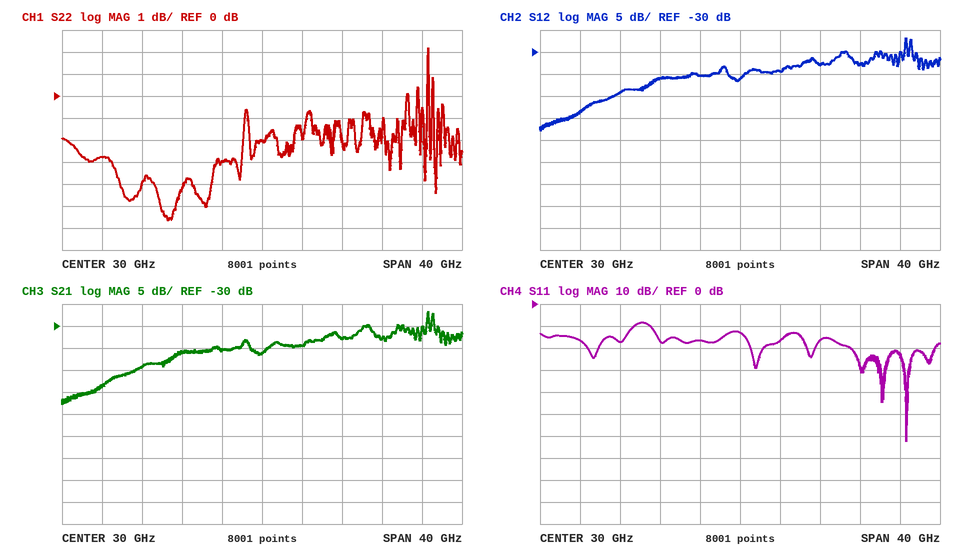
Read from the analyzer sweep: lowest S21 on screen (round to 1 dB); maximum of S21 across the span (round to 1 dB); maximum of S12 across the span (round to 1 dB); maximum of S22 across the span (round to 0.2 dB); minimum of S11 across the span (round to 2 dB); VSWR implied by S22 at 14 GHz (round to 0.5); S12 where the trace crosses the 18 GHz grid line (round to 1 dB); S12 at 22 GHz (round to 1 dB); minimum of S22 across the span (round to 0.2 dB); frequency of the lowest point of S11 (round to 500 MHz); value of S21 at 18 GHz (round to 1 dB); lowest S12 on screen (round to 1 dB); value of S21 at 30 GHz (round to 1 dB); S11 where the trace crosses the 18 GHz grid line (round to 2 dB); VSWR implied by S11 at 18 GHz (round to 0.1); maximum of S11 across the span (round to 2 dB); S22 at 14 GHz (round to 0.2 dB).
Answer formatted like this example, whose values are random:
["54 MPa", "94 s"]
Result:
["-48 dB", "-27 dB", "-27 dB", "2.2 dB", "-62 dB", "6.5", "-39 dB", "-36 dB", "-5.6 dB", "46.5 GHz", "-39 dB", "-48 dB", "-36 dB", "-18 dB", "1.3", "-8 dB", "-2.8 dB"]
